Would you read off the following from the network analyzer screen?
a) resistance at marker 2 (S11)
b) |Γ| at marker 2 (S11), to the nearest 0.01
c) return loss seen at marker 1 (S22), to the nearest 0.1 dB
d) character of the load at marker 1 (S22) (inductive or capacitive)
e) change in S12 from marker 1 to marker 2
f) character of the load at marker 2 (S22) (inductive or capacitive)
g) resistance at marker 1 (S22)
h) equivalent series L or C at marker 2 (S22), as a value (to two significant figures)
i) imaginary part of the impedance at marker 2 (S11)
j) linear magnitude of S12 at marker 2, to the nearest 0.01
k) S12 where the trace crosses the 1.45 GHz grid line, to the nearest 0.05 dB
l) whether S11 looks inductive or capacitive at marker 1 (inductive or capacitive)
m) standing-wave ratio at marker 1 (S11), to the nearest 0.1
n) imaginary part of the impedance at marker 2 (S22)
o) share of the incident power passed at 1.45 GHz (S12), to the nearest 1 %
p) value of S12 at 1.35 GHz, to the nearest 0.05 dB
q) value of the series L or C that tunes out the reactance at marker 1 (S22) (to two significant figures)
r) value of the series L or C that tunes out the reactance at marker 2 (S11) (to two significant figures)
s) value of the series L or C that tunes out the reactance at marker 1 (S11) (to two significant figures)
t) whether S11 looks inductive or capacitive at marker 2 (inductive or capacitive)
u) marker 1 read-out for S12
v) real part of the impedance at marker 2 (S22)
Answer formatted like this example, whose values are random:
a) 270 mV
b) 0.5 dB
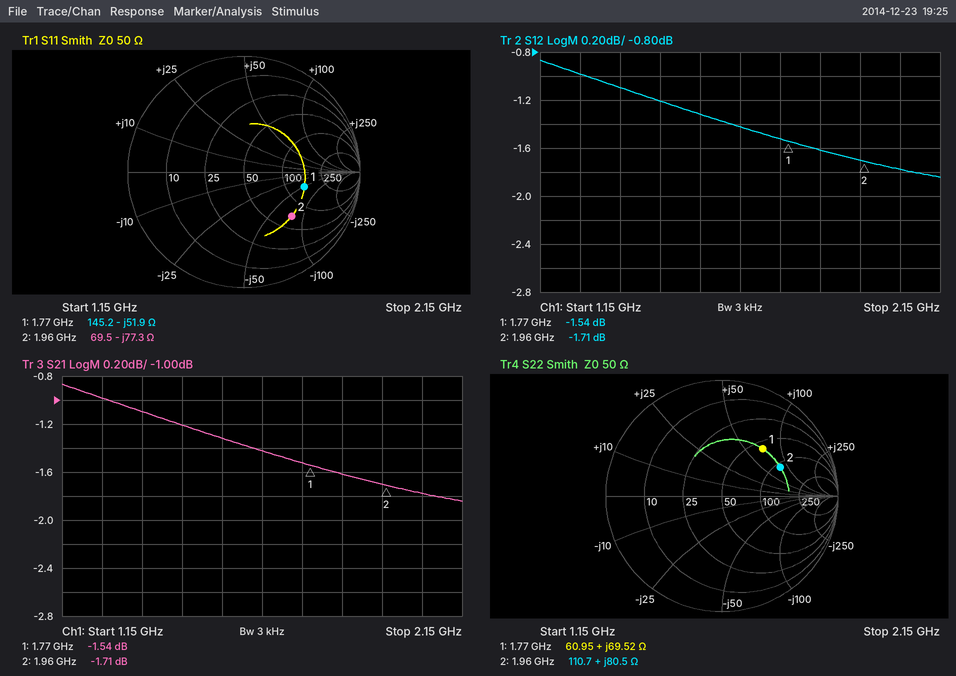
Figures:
a) 69.5 Ω
b) 0.56
c) 5.4 dB
d) inductive
e) -0.17 dB
f) inductive
g) 60.95 Ω
h) 6.5 nH
i) -77.3 Ω
j) 0.82
k) -1.20 dB
l) capacitive
m) 3.3
n) +80.5 Ω
o) 76 %
p) -1.10 dB
q) 1.3 pF
r) 6.3 nH
s) 4.7 nH
t) capacitive
u) -1.54 dB
v) 110.7 Ω
